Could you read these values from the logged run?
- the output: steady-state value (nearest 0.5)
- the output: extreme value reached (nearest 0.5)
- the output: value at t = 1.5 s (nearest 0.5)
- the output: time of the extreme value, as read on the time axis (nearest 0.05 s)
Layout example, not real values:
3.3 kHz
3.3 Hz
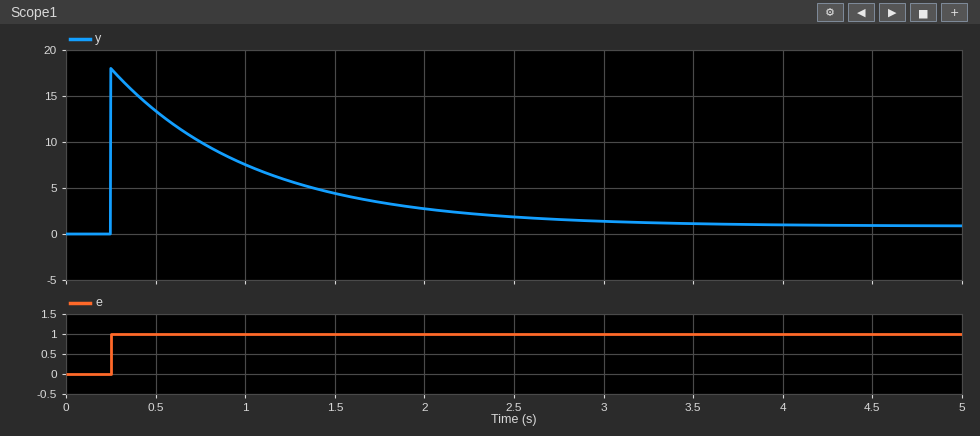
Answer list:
1.0
18.0
4.5
0.25 s
